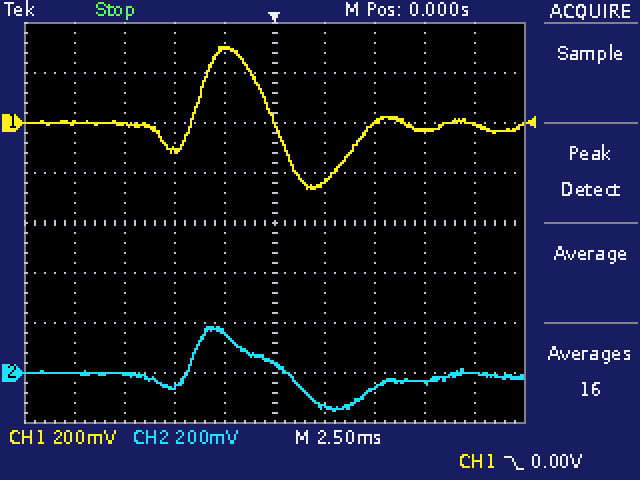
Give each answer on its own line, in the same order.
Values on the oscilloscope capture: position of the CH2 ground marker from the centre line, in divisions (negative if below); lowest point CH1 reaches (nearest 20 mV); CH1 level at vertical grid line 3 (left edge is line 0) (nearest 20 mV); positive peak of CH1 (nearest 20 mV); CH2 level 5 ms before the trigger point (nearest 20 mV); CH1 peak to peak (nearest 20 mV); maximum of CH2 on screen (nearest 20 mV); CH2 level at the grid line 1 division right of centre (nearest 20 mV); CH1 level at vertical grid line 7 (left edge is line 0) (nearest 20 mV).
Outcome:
-3.0 div
-260 mV
-100 mV
300 mV
-60 mV
560 mV
180 mV
-140 mV
0 mV
